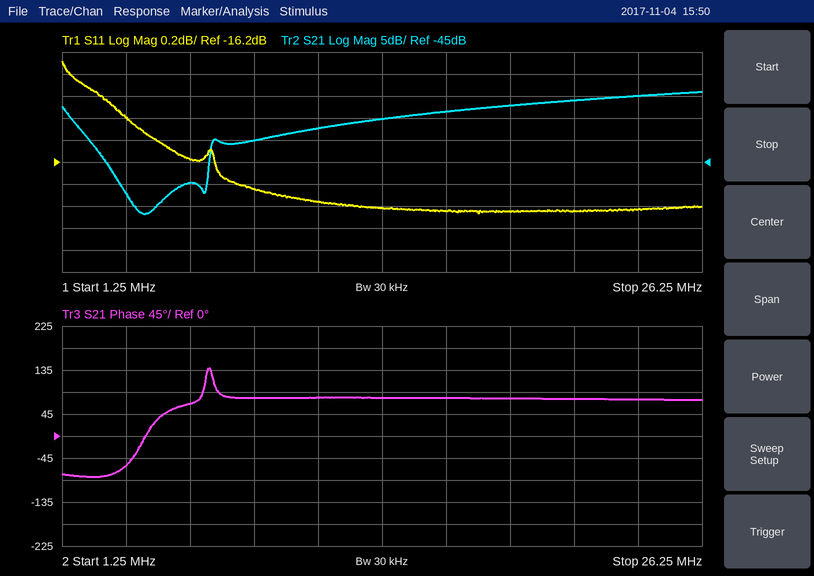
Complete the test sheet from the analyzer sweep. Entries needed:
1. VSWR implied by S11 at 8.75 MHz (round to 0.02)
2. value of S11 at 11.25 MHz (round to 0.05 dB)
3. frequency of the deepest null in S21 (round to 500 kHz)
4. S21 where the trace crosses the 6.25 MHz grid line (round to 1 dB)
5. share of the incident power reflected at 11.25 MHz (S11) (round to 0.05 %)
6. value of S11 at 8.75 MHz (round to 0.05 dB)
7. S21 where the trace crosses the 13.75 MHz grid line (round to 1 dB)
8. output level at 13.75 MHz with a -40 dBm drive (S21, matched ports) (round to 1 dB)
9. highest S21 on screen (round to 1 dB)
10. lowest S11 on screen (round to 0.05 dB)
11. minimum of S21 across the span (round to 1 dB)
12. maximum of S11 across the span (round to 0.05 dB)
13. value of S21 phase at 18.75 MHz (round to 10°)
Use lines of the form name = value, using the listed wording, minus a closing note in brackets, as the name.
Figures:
VSWR implied by S11 at 8.75 MHz = 1.36
value of S11 at 11.25 MHz = -16.55 dB
frequency of the deepest null in S21 = 4.5 MHz
S21 where the trace crosses the 6.25 MHz grid line = -50 dB
share of the incident power reflected at 11.25 MHz (S11) = 2.20 %
value of S11 at 8.75 MHz = -16.45 dB
S21 where the trace crosses the 13.75 MHz grid line = -35 dB
output level at 13.75 MHz with a -40 dBm drive (S21, matched ports) = -75 dBm
highest S21 on screen = -29 dB
lowest S11 on screen = -16.65 dB
minimum of S21 across the span = -57 dB
maximum of S11 across the span = -15.30 dB
value of S21 phase at 18.75 MHz = 80°
